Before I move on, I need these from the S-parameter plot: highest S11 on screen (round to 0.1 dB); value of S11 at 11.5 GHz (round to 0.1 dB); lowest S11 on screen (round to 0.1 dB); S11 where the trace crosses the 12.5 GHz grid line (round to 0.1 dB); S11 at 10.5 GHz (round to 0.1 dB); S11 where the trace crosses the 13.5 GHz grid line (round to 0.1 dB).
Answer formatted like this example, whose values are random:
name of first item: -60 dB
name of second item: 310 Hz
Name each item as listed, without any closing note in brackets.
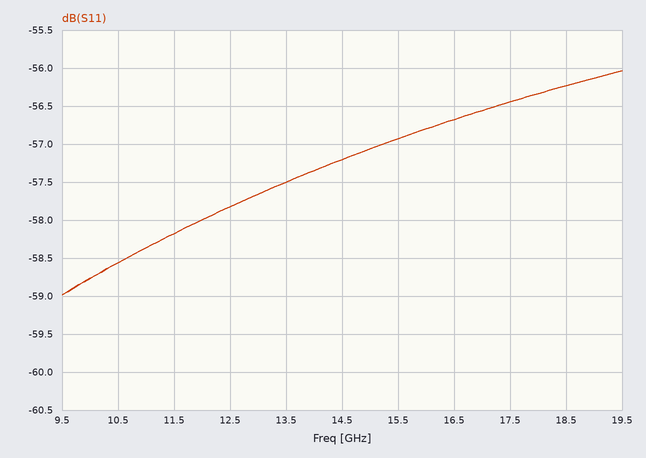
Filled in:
highest S11 on screen: -56.0 dB
value of S11 at 11.5 GHz: -58.2 dB
lowest S11 on screen: -59.0 dB
S11 where the trace crosses the 12.5 GHz grid line: -57.8 dB
S11 at 10.5 GHz: -58.6 dB
S11 where the trace crosses the 13.5 GHz grid line: -57.5 dB
